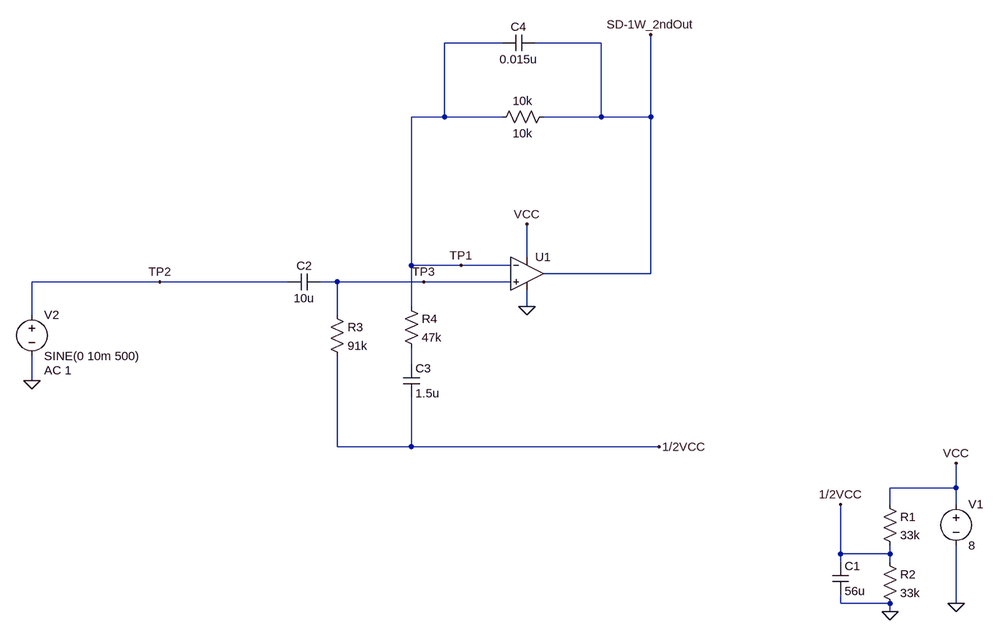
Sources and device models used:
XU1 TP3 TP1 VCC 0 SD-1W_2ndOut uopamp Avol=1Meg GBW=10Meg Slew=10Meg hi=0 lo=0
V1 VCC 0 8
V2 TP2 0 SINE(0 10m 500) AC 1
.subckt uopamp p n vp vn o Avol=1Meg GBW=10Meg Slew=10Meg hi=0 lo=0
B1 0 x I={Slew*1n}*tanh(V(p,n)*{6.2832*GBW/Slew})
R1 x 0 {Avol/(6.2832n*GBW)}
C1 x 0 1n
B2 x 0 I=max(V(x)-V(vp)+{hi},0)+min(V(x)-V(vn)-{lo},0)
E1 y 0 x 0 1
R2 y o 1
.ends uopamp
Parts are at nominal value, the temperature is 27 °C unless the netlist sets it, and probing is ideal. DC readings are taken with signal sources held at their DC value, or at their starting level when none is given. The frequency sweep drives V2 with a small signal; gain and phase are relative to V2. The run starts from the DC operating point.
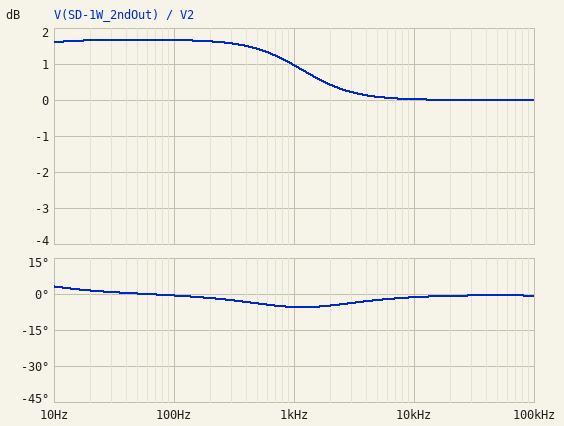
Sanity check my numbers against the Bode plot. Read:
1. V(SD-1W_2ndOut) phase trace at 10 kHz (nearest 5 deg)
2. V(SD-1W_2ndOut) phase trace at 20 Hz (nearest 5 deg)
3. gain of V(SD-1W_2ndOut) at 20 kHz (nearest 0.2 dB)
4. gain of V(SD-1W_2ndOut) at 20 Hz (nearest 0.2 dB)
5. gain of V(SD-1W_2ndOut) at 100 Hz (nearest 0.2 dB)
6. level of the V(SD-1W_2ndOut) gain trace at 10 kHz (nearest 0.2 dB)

0 deg
0 deg
0 dB
1.6 dB
1.6 dB
0 dB
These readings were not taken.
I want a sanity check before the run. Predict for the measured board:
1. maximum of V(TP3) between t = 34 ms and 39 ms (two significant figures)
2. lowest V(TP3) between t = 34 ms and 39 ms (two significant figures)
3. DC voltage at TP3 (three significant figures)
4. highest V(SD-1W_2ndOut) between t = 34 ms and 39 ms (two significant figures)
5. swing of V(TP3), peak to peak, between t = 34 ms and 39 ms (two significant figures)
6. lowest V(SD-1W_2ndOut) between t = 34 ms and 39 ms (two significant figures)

4.0 V
4.0 V
4.00 V
4.0 V
20 mV
4.0 V
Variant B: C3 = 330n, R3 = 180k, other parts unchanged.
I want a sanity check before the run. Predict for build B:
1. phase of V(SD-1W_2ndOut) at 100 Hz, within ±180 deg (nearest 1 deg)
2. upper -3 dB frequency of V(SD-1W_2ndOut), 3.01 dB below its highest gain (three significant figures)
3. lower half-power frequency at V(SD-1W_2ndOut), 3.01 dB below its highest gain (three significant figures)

0 deg
6.04 MHz
148 mHz
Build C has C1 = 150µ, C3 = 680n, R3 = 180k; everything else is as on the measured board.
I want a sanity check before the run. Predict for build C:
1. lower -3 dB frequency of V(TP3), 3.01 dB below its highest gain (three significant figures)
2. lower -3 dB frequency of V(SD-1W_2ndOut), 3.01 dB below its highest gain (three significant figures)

88.9 mHz
152 mHz
